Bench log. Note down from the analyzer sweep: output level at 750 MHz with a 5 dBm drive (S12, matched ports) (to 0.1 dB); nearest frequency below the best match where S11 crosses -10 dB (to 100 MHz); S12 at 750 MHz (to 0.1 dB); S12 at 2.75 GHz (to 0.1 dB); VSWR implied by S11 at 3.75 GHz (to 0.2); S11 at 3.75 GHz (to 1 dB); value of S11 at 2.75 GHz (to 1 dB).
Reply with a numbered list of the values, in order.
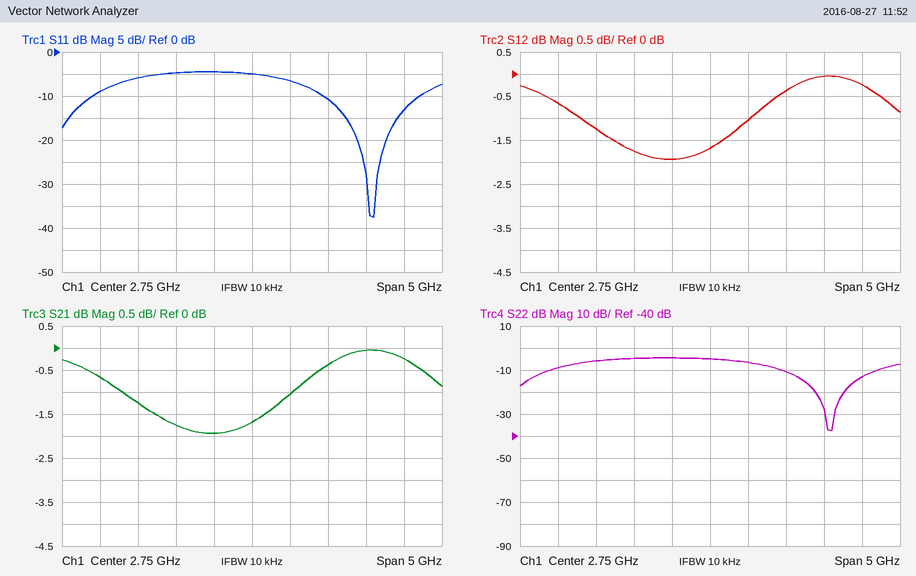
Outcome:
1. 4.3 dBm
2. 3.7 GHz
3. -0.7 dB
4. -1.7 dB
5. 1.8
6. -11 dB
7. -5 dB
